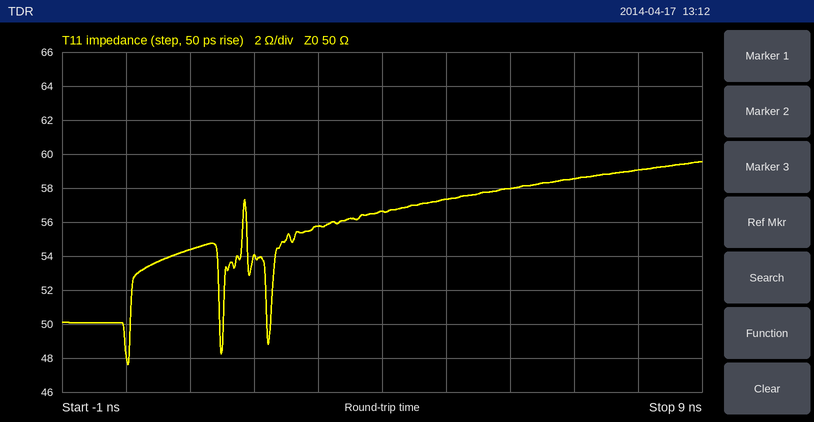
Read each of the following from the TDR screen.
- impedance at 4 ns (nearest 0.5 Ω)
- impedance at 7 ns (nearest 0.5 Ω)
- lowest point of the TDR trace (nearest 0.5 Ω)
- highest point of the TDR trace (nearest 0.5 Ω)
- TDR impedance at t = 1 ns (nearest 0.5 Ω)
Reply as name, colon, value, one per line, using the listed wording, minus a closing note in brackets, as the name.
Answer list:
impedance at 4 ns: 56.5 Ω
impedance at 7 ns: 58.5 Ω
lowest point of the TDR trace: 47.5 Ω
highest point of the TDR trace: 59.5 Ω
TDR impedance at t = 1 ns: 54.5 Ω
